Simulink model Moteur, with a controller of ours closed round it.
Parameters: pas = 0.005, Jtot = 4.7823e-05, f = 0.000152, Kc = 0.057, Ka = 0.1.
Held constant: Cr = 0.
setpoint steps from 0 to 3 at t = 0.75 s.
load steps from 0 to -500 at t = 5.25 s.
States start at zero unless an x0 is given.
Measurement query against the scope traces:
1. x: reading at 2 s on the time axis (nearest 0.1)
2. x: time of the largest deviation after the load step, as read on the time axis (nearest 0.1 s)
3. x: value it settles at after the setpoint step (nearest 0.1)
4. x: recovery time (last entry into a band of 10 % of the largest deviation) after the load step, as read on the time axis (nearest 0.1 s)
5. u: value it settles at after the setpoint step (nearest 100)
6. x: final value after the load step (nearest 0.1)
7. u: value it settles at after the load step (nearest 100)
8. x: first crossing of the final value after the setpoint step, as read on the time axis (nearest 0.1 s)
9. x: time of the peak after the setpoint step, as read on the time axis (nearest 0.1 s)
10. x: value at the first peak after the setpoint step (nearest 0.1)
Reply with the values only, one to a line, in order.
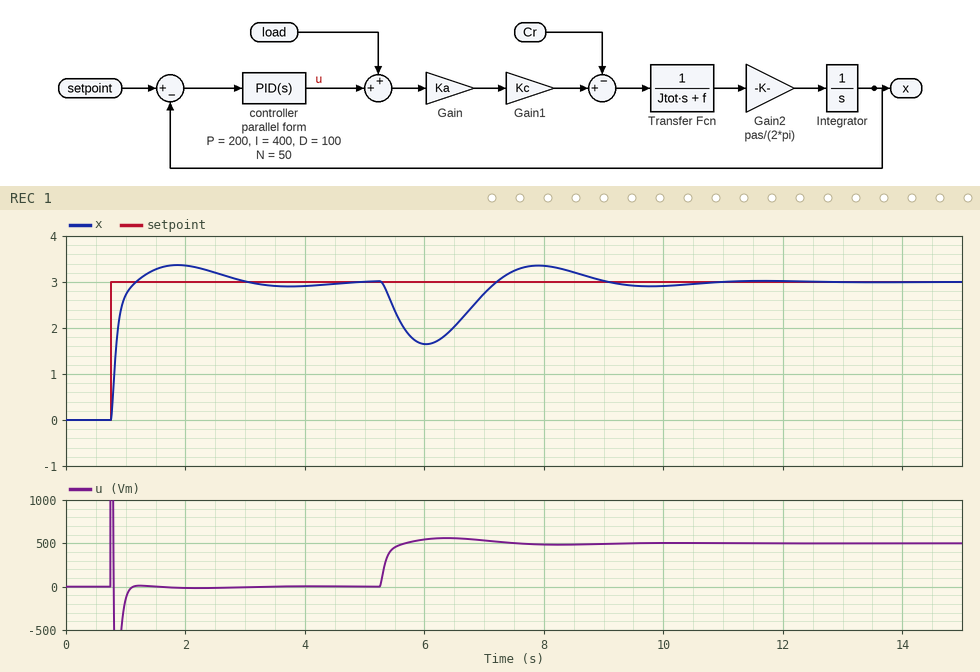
3.4
6.0 s
3.0
8.7 s
0
3.0
500
1.2 s
1.9 s
3.4
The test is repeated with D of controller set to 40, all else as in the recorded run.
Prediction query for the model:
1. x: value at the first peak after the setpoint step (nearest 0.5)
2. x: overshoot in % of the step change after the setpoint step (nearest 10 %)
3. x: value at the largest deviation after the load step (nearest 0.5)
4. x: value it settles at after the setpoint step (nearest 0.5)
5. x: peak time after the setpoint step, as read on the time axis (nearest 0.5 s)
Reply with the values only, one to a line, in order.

4.0
30 %
1.0
3.0
1.5 s
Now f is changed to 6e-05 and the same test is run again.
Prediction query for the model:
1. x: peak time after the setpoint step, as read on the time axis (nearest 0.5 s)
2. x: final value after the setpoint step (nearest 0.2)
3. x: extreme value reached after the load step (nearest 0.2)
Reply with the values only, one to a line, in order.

1.5 s
3.0
1.6
